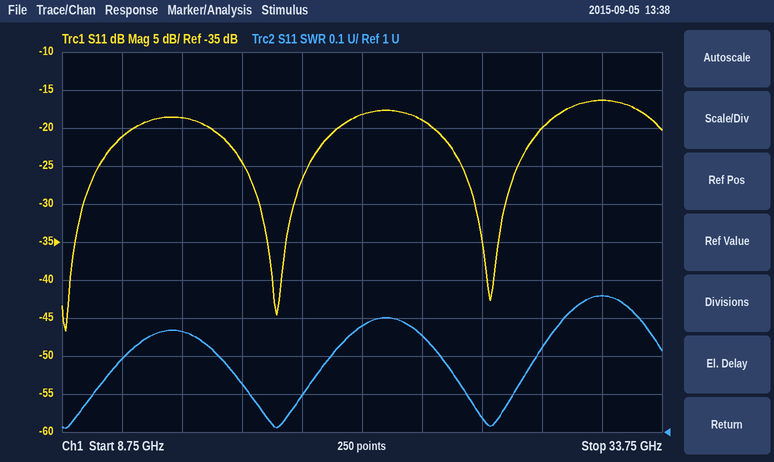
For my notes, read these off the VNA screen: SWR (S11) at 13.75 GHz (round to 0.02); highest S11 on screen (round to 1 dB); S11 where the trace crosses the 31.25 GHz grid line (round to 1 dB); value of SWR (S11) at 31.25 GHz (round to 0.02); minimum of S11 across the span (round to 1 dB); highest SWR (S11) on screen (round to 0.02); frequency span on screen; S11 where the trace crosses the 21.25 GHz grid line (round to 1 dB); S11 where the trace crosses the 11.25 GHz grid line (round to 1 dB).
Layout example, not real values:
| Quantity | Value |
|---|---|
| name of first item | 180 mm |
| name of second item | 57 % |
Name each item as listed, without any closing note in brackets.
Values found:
| Quantity | Value |
|---|---|
| SWR (S11) at 13.75 GHz | 1.26 |
| highest S11 on screen | -16 dB |
| S11 where the trace crosses the 31.25 GHz grid line | -16 dB |
| value of SWR (S11) at 31.25 GHz | 1.36 |
| minimum of S11 across the span | -47 dB |
| highest SWR (S11) on screen | 1.36 |
| frequency span on screen | 25 GHz |
| S11 where the trace crosses the 21.25 GHz grid line | -18 dB |
| S11 where the trace crosses the 11.25 GHz grid line | -21 dB |
